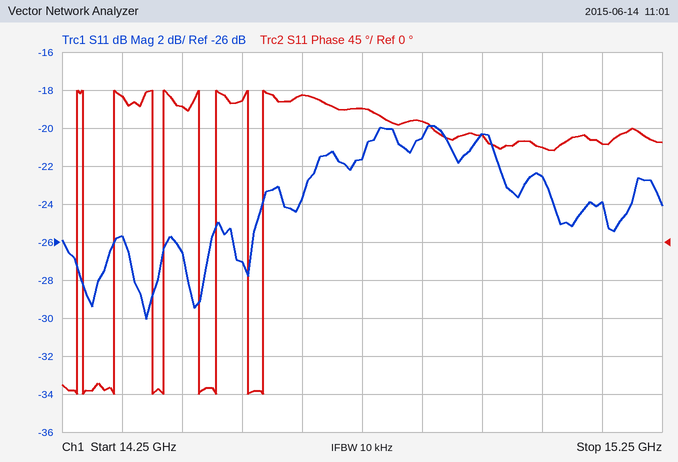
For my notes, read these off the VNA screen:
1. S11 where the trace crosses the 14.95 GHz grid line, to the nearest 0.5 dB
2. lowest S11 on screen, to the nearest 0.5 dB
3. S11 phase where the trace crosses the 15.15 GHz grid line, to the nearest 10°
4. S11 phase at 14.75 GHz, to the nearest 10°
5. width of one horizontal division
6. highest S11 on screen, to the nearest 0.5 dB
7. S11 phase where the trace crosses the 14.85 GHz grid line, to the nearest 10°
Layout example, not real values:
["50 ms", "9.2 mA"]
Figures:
["-20.5 dB", "-30.0 dB", "120°", "160°", "100 MHz", "-20.0 dB", "140°"]
